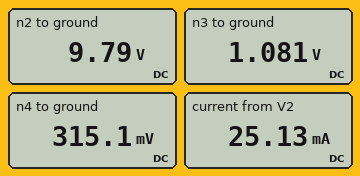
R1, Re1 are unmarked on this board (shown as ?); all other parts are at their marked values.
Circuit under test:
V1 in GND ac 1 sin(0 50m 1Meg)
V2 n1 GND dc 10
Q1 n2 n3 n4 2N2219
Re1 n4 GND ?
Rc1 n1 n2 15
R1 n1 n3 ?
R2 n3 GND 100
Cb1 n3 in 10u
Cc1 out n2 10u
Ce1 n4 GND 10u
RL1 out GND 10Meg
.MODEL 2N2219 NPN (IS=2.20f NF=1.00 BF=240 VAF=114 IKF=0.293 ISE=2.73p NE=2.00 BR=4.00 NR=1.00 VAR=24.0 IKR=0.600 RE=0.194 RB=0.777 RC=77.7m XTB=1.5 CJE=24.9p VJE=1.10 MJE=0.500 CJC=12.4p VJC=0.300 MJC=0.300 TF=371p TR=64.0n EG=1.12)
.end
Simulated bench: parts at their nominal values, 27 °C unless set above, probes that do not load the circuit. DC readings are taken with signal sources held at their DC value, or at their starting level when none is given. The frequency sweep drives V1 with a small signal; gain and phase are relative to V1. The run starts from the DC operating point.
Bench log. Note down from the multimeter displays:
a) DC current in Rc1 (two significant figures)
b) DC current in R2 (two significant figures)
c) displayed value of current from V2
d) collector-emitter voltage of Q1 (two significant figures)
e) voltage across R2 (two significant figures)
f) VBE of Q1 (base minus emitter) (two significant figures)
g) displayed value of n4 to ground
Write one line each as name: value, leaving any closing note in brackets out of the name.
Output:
DC current in Rc1: 14 mA
DC current in R2: 11 mA
displayed value of current from V2: 25.13 mA
collector-emitter voltage of Q1: 9.5 V
voltage across R2: 1.1 V
VBE of Q1 (base minus emitter): 770 mV
displayed value of n4 to ground: 315.1 mV
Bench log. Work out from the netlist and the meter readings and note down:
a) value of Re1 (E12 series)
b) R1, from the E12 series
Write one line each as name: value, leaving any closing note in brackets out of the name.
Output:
value of Re1: 22 Ω
R1, from the E12 series: 820 Ω
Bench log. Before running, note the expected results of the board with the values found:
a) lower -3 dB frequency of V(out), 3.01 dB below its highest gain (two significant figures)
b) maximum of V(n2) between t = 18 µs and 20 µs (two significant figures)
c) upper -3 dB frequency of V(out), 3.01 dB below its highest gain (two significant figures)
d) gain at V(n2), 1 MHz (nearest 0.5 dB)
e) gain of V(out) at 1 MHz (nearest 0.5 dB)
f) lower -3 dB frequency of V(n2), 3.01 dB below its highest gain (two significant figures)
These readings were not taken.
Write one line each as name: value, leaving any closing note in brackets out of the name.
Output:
lower -3 dB frequency of V(out), 3.01 dB below its highest gain: 8.3 kHz
maximum of V(n2) between t = 18 µs and 20 µs: 10 V
upper -3 dB frequency of V(out), 3.01 dB below its highest gain: 620 MHz
gain at V(n2), 1 MHz: 17.0 dB
gain of V(out) at 1 MHz: 17.0 dB
lower -3 dB frequency of V(n2), 3.01 dB below its highest gain: 8.3 kHz
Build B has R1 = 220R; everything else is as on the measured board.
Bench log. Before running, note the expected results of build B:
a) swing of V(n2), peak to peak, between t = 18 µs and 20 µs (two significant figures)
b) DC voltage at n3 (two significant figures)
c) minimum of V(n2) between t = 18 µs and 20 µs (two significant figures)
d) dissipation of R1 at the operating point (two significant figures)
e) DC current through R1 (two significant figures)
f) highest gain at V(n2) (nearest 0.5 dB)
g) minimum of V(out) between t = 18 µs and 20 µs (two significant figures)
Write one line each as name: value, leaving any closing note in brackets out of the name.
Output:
swing of V(n2), peak to peak, between t = 18 µs and 20 µs: 2.6 V
DC voltage at n3: 3.1 V
minimum of V(n2) between t = 18 µs and 20 µs: 7.0 V
dissipation of R1 at the operating point: 220 mW
DC current through R1: 31 mA
highest gain at V(n2): 29.0 dB
minimum of V(out) between t = 18 µs and 20 µs: -1.5 V
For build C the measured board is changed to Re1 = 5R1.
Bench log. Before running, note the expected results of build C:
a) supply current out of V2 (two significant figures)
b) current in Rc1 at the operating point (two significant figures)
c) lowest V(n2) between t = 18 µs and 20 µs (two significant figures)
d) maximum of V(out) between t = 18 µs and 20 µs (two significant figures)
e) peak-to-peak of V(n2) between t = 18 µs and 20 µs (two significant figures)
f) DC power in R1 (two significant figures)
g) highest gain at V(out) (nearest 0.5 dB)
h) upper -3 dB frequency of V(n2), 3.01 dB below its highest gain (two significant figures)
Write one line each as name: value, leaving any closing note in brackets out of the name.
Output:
supply current out of V2: 61 mA
current in Rc1 at the operating point: 50 mA
lowest V(n2) between t = 18 µs and 20 µs: 8.2 V
maximum of V(out) between t = 18 µs and 20 µs: 630 mV
peak-to-peak of V(n2) between t = 18 µs and 20 µs: 1.7 V
DC power in R1: 97 mW
highest gain at V(out): 25.5 dB
upper -3 dB frequency of V(n2), 3.01 dB below its highest gain: 280 MHz
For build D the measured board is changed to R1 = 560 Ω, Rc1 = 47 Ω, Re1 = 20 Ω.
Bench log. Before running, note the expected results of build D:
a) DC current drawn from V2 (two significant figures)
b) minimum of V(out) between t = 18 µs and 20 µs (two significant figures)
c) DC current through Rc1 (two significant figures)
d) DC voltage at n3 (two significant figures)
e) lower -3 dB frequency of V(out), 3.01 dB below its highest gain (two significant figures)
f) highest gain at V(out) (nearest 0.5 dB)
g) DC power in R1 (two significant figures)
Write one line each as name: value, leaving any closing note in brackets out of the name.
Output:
DC current drawn from V2: 50 mA
minimum of V(out) between t = 18 µs and 20 µs: -2.6 V
DC current through Rc1: 35 mA
DC voltage at n3: 1.5 V
lower -3 dB frequency of V(out), 3.01 dB below its highest gain: 16 kHz
highest gain at V(out): 33.0 dB
DC power in R1: 130 mW
